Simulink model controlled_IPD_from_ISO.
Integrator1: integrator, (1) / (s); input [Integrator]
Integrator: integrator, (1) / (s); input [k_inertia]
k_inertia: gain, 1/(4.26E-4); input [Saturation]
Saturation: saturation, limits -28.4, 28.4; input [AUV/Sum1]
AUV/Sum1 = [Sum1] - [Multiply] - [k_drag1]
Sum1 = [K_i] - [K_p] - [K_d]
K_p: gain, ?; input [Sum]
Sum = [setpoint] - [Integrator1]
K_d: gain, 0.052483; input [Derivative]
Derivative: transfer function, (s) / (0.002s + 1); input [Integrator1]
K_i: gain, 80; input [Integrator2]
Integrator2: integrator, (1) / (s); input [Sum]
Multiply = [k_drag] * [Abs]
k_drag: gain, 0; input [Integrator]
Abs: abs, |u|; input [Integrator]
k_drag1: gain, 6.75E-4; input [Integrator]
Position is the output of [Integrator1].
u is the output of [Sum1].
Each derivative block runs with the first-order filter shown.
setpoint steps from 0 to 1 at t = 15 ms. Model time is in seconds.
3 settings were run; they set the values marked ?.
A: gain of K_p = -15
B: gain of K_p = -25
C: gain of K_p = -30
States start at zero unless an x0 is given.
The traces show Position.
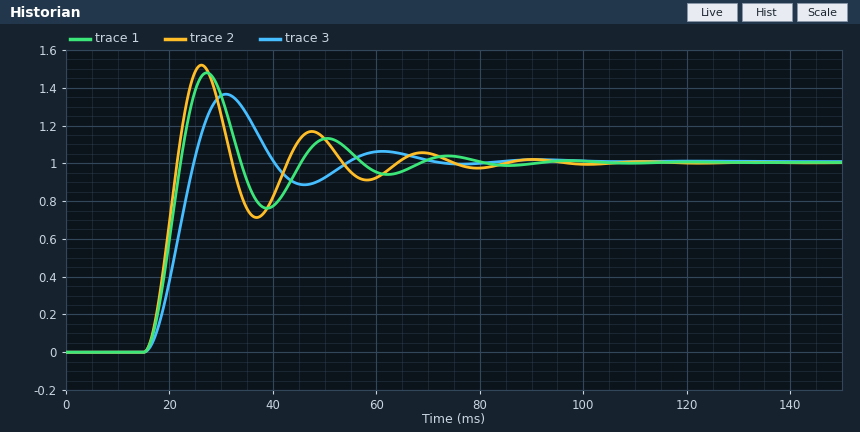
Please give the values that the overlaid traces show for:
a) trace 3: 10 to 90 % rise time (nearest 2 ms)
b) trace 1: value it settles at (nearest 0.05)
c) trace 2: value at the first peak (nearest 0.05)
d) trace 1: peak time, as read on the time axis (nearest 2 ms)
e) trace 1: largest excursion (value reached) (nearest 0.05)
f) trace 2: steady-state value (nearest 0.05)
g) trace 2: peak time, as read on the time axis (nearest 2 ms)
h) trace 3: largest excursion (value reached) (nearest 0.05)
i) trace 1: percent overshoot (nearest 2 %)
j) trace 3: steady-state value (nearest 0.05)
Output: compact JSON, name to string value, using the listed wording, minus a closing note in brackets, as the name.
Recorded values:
{"trace 3: 10 to 90 % rise time": "6 ms", "trace 1: value it settles at": "1.00", "trace 2: value at the first peak": "1.50", "trace 1: peak time, as read on the time axis": "28 ms", "trace 1: largest excursion (value reached)": "1.50", "trace 2: steady-state value": "1.00", "trace 2: peak time, as read on the time axis": "26 ms", "trace 3: largest excursion (value reached)": "1.35", "trace 1: percent overshoot": "48 %", "trace 3: steady-state value": "1.00"}
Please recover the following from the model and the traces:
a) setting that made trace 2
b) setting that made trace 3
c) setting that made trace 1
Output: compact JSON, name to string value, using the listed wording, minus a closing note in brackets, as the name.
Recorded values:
{"setting that made trace 2": "C", "setting that made trace 3": "A", "setting that made trace 1": "B"}
